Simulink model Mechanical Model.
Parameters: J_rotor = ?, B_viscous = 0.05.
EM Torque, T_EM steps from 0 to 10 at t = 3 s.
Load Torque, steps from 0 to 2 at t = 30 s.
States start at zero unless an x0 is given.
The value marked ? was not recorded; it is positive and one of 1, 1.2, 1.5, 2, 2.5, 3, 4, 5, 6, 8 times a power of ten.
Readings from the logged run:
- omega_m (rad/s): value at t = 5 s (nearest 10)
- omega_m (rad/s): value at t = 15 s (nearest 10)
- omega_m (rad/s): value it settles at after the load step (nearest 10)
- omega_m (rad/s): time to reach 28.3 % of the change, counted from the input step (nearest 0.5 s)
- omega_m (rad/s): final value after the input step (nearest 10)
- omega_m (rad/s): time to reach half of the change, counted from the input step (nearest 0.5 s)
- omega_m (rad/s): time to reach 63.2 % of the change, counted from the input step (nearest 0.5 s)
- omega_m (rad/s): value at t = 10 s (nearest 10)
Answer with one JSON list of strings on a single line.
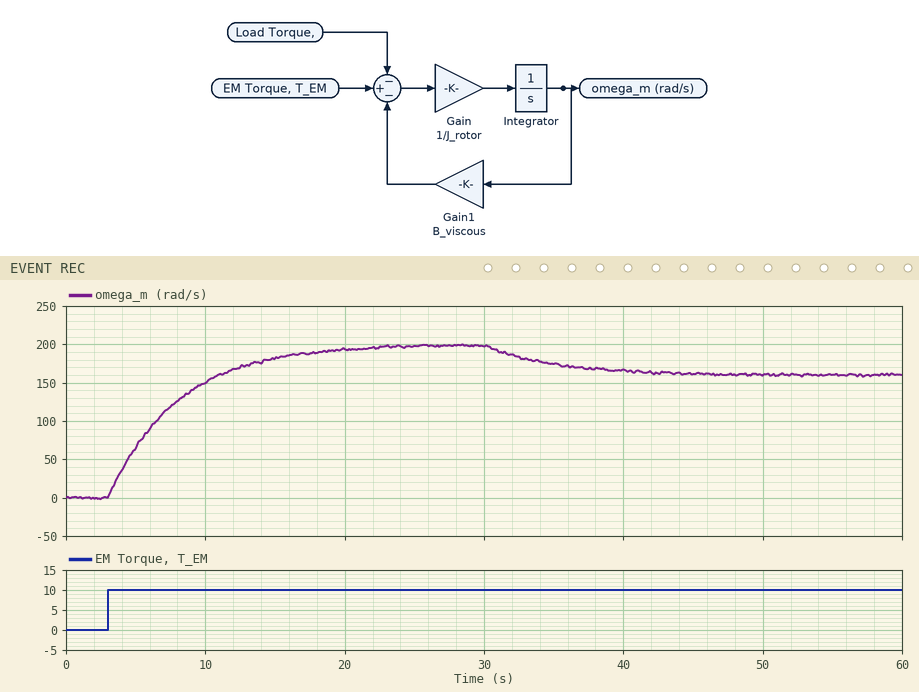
["70", "180", "160", "1.5 s", "200", "3.5 s", "5.0 s", "150"]
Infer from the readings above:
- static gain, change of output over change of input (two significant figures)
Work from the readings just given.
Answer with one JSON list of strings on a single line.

["20"]
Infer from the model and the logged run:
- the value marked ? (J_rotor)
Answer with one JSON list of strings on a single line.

["0.25"]
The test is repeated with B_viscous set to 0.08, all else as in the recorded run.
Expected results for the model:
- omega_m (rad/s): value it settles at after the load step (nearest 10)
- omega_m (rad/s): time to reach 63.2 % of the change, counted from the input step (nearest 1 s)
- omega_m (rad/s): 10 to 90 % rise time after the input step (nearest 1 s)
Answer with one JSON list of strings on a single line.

["100", "3 s", "7 s"]
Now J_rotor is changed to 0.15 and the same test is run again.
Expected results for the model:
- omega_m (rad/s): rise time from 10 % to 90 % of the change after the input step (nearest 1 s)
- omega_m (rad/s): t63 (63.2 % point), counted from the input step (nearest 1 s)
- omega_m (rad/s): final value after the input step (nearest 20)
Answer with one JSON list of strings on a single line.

["7 s", "3 s", "200"]
